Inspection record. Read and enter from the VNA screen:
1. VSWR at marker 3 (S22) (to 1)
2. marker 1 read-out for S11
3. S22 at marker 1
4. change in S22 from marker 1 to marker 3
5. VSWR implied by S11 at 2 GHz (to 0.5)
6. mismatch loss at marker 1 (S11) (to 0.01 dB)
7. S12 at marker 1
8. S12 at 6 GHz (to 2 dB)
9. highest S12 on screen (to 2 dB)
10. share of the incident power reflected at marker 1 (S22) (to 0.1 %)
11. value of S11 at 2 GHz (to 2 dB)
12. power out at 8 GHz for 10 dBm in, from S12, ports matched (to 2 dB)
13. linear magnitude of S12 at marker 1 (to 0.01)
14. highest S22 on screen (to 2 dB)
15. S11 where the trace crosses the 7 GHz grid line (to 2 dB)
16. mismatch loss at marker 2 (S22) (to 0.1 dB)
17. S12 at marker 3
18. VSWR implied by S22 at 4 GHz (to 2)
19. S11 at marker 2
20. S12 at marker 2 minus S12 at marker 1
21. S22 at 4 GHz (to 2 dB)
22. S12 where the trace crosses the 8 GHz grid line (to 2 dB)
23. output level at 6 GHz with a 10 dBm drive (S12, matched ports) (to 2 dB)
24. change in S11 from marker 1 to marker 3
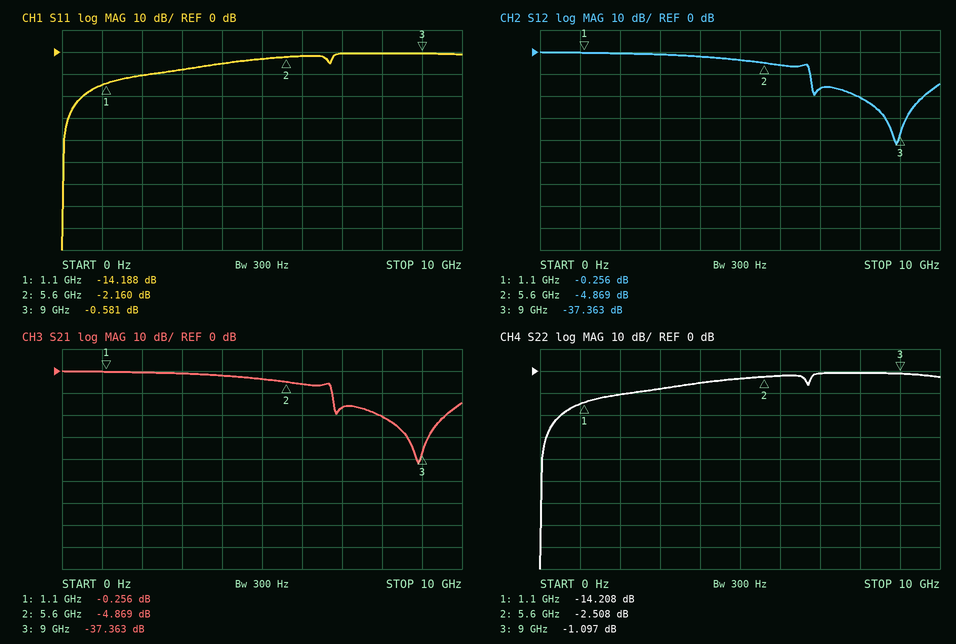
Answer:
16
-14.188 dB
-14.208 dB
13.111 dB
2.0
0.17 dB
-0.256 dB
-6 dB
0 dB
3.8 %
-10 dB
-10 dBm
0.97
0 dB
0 dB
3.6 dB
-37.363 dB
4
-2.160 dB
-4.613 dB
-6 dB
-20 dB
4 dBm
13.607 dB
